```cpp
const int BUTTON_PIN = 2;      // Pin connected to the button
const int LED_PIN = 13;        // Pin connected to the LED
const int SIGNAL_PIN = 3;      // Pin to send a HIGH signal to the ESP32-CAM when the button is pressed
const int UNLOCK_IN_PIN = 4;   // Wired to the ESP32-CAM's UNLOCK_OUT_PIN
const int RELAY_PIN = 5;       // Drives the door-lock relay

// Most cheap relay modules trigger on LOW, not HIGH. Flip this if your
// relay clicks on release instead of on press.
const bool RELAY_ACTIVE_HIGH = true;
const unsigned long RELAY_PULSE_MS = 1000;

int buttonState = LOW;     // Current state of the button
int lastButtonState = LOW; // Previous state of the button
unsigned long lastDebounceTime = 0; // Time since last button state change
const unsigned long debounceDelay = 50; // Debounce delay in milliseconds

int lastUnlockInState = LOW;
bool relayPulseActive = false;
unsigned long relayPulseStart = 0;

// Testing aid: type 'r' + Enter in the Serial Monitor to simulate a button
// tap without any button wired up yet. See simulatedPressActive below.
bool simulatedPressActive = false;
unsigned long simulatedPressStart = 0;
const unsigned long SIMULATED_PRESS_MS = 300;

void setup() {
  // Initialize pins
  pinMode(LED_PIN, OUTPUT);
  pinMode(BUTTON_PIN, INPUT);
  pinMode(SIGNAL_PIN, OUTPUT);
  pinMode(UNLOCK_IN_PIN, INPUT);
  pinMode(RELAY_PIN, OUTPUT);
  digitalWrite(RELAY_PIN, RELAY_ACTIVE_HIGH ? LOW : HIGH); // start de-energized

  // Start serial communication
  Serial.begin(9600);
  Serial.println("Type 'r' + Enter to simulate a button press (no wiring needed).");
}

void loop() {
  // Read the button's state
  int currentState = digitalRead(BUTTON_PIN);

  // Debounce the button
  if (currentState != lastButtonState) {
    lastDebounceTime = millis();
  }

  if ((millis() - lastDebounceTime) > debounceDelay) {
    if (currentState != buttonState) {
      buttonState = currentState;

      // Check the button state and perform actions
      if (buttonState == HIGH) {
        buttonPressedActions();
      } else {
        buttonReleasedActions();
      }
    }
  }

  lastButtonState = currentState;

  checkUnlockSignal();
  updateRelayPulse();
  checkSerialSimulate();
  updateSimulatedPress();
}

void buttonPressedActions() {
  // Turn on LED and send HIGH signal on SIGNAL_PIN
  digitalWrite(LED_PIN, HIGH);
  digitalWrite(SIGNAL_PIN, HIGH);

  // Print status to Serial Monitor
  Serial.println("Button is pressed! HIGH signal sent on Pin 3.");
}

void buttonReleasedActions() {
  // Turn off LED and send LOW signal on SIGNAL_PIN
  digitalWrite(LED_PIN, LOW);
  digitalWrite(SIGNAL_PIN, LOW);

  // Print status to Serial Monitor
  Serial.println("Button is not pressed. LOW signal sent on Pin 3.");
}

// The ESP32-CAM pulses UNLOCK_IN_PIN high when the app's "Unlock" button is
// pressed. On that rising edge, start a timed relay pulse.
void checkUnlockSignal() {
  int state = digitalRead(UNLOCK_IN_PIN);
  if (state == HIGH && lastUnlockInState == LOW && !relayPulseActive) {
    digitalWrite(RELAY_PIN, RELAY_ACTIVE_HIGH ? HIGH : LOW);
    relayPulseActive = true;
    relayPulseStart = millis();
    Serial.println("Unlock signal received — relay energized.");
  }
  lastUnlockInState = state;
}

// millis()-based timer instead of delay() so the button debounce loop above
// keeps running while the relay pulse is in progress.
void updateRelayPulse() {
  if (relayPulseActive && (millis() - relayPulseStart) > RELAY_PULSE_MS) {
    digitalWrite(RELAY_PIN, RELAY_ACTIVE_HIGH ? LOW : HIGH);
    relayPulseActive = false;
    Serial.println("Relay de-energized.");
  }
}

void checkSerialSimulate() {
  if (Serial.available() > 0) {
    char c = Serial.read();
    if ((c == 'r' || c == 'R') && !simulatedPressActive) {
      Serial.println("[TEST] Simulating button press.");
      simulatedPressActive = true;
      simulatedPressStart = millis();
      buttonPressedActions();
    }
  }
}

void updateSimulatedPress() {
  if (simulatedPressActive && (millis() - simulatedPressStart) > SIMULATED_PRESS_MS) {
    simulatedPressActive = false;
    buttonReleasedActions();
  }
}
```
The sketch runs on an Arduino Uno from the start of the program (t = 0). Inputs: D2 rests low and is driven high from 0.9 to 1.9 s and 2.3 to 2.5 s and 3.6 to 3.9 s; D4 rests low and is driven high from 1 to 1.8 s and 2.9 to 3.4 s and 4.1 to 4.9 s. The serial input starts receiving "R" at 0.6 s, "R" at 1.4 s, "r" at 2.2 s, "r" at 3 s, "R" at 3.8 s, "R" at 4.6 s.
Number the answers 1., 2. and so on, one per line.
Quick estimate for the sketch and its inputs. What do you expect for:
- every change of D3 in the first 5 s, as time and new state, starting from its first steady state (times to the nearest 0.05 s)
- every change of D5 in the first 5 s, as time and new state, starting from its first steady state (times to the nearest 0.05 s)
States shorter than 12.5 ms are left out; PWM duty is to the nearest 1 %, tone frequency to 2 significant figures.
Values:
1. 0 s low; 0.6 s high; 0.9 s low; 0.95 s high; 1.7 s low; 2.2 s high; 2.5 s low; 3 s high; 3.3 s low; 3.65 s high; 3.95 s low; 4.6 s high; 4.9 s low
2. 0 s low; 1 s high; 2 s low; 2.9 s high; 3.9 s low; 4.1 s high
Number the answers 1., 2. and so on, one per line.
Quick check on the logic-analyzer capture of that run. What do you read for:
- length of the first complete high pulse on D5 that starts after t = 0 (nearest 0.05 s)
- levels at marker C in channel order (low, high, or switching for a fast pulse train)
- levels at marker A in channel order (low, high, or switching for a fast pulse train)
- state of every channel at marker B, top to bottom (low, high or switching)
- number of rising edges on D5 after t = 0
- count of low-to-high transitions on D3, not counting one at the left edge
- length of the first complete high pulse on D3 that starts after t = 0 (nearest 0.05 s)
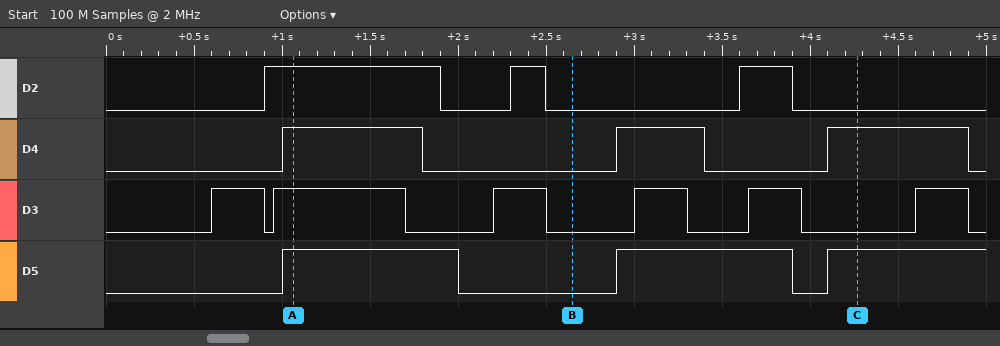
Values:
1. 1.00 s
2. D2 low, D4 high, D3 low, D5 high
3. D2 high, D4 high, D3 high, D5 high
4. D2 low, D4 low, D3 low, D5 low
5. 3
6. 6
7. 0.30 s
